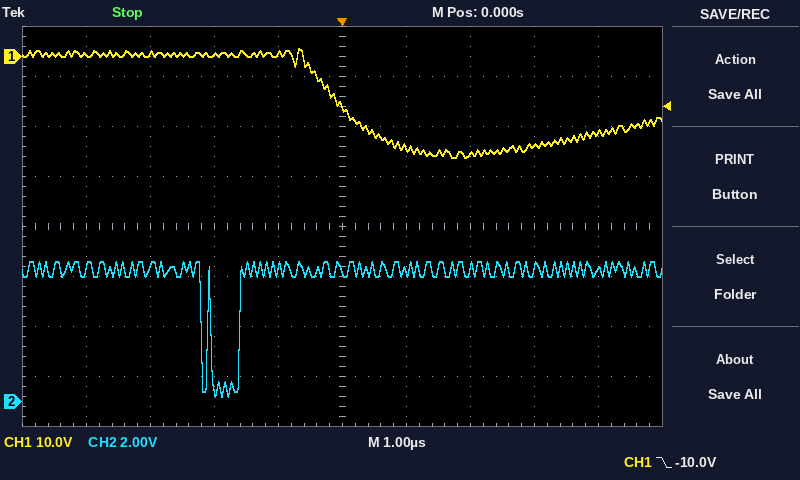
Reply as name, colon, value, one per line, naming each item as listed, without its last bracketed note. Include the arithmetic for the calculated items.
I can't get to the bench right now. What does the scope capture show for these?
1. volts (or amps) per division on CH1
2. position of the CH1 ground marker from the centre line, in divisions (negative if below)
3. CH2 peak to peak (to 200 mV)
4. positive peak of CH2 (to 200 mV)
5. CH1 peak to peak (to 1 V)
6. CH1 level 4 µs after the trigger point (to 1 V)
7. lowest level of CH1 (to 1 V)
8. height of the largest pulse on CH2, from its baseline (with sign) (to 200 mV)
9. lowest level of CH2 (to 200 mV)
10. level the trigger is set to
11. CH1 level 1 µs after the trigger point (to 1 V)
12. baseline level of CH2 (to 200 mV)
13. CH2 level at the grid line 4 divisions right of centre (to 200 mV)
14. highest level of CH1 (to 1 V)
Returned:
volts (or amps) per division on CH1: 10 V
position of the CH1 ground marker from the centre line, in divisions: +3.4 div
CH2 peak to peak: 5.6 V − (200 mV) = 5.4 V
positive peak of CH2: 5.6 V
CH1 peak to peak: 2 V − (-20 V) = 22 V
CH1 level 4 µs after the trigger point: -15 V
lowest level of CH1: -20 V
height of the largest pulse on CH2, from its baseline (with sign): 200 mV − (5.2 V) = -5.0 V
lowest level of CH2: 200 mV
level the trigger is set to: -10.0 V
CH1 level 1 µs after the trigger point: -18 V
baseline level of CH2: 5.2 V
CH2 level at the grid line 4 divisions right of centre: 5.2 V
highest level of CH1: 2 V
